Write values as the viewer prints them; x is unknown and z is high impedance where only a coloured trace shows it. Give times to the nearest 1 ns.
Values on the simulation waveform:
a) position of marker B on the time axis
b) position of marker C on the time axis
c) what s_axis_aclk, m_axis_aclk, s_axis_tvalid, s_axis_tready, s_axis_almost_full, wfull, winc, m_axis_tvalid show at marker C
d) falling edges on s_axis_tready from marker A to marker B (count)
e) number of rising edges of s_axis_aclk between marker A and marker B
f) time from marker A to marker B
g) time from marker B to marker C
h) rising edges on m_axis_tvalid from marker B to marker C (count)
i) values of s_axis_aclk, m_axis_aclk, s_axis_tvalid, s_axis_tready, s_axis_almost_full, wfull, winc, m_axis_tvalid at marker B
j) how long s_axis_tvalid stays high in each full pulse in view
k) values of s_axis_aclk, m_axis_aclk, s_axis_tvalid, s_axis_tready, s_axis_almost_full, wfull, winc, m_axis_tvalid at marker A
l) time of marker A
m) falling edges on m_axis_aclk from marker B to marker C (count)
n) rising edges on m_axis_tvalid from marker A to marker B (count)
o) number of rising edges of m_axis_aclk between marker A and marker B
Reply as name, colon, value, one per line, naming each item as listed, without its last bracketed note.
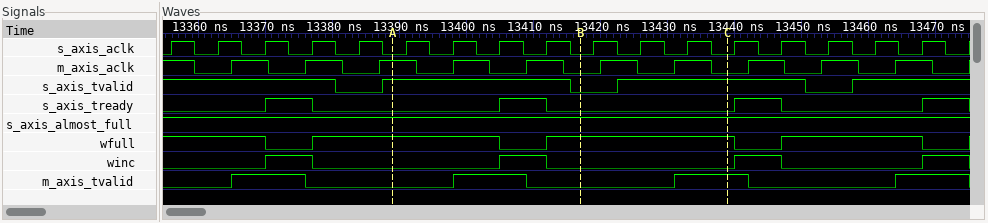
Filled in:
position of marker B on the time axis: 13417 ns
position of marker C on the time axis: 13439 ns
what s_axis_aclk, m_axis_aclk, s_axis_tvalid, s_axis_tready, s_axis_almost_full, wfull, winc, m_axis_tvalid show at marker C: s_axis_aclk=0, m_axis_aclk=0, s_axis_tvalid=1, s_axis_tready=0, s_axis_almost_full=1, wfull=1, winc=0, m_axis_tvalid=1
falling edges on s_axis_tready from marker A to marker B: 1
number of rising edges of s_axis_aclk between marker A and marker B: 4
time from marker A to marker B: 28 ns
time from marker B to marker C: 22 ns
rising edges on m_axis_tvalid from marker B to marker C: 1
values of s_axis_aclk, m_axis_aclk, s_axis_tvalid, s_axis_tready, s_axis_almost_full, wfull, winc, m_axis_tvalid at marker B: s_axis_aclk=0, m_axis_aclk=0, s_axis_tvalid=0, s_axis_tready=0, s_axis_almost_full=1, wfull=1, winc=0, m_axis_tvalid=0
how long s_axis_tvalid stays high in each full pulse in view: 28 ns, 28 ns
values of s_axis_aclk, m_axis_aclk, s_axis_tvalid, s_axis_tready, s_axis_almost_full, wfull, winc, m_axis_tvalid at marker A: s_axis_aclk=0, m_axis_aclk=1, s_axis_tvalid=1, s_axis_tready=0, s_axis_almost_full=1, wfull=1, winc=0, m_axis_tvalid=0
time of marker A: 13389 ns
falling edges on m_axis_aclk from marker B to marker C: 2
rising edges on m_axis_tvalid from marker A to marker B: 1
number of rising edges of m_axis_aclk between marker A and marker B: 2
